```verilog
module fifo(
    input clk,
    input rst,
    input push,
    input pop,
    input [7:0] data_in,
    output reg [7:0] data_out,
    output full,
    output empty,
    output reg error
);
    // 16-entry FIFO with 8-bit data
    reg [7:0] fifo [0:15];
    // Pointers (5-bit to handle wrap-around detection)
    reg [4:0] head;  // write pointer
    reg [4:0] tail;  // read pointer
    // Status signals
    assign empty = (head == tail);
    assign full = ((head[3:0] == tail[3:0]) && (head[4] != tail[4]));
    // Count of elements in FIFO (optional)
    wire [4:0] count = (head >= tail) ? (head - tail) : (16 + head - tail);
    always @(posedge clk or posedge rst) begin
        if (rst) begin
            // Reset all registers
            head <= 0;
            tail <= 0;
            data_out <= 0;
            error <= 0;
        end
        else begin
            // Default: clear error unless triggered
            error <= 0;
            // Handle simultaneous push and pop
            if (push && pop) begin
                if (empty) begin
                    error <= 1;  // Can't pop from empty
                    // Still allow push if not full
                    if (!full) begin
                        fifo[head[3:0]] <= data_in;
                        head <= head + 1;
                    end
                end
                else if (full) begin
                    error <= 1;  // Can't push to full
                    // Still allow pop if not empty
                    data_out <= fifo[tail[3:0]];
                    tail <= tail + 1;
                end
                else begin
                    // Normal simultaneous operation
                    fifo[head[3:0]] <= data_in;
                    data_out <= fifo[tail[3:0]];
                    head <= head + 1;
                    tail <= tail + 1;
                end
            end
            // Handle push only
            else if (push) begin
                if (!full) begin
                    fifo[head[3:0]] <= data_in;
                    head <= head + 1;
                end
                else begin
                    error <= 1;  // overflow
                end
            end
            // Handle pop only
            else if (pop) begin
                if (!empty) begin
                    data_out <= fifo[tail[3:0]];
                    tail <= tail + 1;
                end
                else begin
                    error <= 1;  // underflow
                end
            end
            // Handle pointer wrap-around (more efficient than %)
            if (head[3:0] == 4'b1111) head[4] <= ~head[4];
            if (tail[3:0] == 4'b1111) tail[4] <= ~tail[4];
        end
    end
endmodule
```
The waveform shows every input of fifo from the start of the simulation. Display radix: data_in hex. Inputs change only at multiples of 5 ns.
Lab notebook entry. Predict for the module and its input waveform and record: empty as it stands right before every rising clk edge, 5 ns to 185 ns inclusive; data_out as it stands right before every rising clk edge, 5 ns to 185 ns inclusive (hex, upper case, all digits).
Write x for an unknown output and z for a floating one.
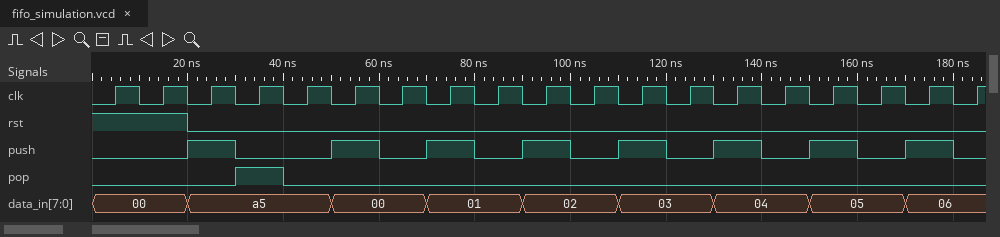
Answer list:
1 1 1 0 1 1 0 0 0 0 0 0 0 0 0 0 0 0 0
00, 00, 00, 00, A5, A5, A5, A5, A5, A5, A5, A5, A5, A5, A5, A5, A5, A5, A5
